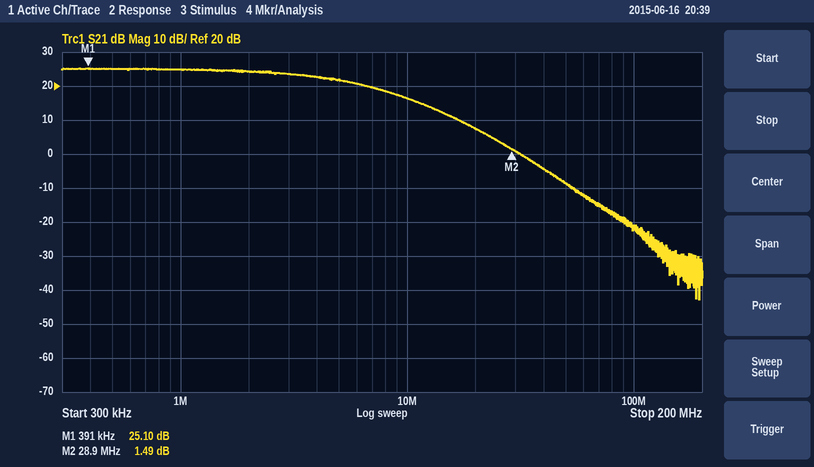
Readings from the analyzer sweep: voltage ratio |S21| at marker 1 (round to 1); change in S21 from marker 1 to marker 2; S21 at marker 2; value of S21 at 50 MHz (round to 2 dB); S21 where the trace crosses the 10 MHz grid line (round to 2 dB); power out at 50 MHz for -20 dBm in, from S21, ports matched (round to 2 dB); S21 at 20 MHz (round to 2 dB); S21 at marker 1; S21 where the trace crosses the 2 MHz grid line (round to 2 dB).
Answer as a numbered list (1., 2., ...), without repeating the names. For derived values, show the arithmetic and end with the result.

1. 10^(25.1/20) ≈ 18
2. 1.49 − (25.1) = -23.61 dB
3. 1.49 dB
4. -8 dB
5. 16 dB
6. -20 dBm + (-8 dB) = -28 dBm
7. 8 dB
8. 25.10 dB
9. 24 dB
